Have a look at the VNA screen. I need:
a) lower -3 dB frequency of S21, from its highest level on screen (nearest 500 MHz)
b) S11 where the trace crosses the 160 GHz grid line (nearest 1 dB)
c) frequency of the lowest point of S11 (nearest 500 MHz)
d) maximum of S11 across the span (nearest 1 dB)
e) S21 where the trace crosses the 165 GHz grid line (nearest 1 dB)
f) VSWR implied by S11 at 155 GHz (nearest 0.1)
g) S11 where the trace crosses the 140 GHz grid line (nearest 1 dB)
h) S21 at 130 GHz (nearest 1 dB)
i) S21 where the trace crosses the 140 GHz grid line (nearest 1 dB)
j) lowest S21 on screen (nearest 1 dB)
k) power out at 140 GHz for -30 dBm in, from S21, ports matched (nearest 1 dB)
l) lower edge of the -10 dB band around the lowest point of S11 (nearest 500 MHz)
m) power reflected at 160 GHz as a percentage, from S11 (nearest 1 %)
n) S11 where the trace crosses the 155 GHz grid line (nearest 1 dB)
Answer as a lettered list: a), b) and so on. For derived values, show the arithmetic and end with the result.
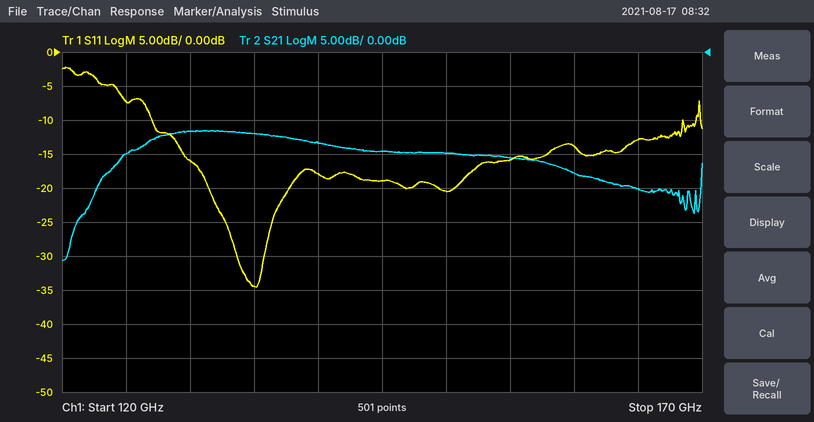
a) 125.5 GHz
b) -14 dB
c) 135.0 GHz
d) -2 dB
e) -20 dB
f) |Γ| = 10^(-16/20) = 0.1585; VSWR = (1 + 0.1585)/(1 − 0.1585) ≈ 1.4
g) -18 dB
h) -12 dB
i) -13 dB
j) -31 dB
k) -30 dBm + (-13 dB) = -43 dBm
l) 127.0 GHz
m) 10^(-14/10) ≈ 4 %
n) -16 dB
